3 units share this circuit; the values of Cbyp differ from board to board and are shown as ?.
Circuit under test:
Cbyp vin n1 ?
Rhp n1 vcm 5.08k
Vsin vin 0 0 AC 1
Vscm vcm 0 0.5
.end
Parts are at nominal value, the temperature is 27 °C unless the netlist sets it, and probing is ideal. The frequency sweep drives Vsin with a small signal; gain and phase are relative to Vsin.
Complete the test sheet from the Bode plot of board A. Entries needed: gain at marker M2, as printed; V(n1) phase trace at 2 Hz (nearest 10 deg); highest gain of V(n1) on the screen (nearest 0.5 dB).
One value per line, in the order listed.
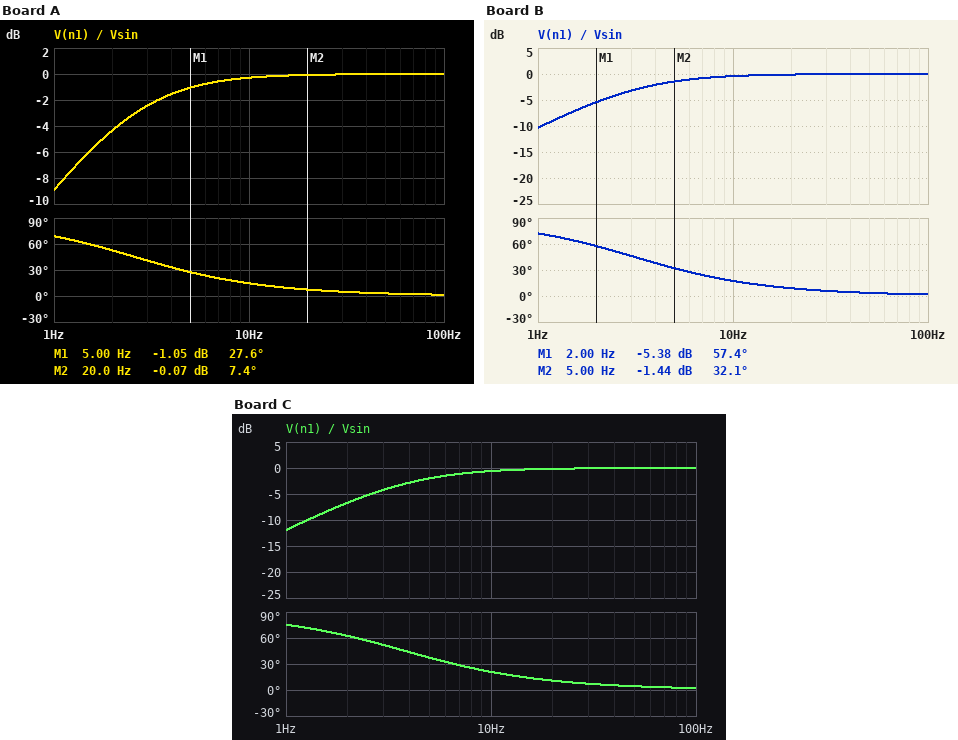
-0.07 dB
50 deg
0 dB
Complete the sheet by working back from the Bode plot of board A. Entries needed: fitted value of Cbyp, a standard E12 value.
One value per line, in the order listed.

12 µF
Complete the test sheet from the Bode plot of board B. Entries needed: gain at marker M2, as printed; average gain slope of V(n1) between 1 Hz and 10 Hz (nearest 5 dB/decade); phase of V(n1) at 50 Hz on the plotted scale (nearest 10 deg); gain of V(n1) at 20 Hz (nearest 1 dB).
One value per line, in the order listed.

-1.44 dB
10 dB/decade
0 deg
0 dB
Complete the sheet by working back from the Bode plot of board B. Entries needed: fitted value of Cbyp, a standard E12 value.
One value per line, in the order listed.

10 µF
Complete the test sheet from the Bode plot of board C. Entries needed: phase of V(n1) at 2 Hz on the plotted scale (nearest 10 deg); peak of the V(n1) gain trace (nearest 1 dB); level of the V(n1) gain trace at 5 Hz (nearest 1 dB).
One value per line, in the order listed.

60 deg
0 dB
-2 dB
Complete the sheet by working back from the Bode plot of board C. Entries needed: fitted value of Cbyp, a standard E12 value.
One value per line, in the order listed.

8.2 µF
